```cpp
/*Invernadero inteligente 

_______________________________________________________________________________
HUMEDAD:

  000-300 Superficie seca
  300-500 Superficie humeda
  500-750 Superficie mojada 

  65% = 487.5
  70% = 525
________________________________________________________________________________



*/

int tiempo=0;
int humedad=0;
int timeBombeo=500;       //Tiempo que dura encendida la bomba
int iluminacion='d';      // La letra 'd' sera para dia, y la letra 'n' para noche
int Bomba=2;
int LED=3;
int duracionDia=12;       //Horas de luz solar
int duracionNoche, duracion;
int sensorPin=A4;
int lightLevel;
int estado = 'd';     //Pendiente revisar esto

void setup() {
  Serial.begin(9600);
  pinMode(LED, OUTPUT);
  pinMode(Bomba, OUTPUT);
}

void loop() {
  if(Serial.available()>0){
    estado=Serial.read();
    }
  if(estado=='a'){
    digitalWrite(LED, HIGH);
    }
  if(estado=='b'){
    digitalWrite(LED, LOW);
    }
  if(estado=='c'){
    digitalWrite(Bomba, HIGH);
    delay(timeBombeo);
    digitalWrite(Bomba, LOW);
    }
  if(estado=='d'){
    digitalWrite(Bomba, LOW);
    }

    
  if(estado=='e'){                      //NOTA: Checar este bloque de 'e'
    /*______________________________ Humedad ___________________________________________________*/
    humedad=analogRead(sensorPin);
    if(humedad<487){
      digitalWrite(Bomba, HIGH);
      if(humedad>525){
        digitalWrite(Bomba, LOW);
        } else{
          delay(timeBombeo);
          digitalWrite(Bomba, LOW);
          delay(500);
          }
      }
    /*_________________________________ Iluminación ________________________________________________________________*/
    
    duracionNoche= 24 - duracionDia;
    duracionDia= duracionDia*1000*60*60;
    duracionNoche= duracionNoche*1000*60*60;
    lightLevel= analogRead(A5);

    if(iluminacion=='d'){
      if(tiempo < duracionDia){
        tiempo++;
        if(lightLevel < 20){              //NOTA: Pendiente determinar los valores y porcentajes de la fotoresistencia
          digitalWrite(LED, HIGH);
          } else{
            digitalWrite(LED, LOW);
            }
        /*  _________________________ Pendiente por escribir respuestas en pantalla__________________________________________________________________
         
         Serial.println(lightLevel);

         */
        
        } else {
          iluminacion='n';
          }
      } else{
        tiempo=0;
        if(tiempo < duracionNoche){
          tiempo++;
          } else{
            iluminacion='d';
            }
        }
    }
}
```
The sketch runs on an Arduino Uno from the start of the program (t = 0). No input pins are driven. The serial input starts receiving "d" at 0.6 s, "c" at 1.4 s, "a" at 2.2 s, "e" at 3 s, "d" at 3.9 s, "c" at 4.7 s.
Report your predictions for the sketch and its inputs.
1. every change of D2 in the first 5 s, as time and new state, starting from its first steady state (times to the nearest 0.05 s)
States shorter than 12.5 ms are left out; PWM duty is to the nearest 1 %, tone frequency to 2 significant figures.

0 s low; 1.4 s high; 2.4 s low; 3 s high; 3.5 s low; 4.7 s high
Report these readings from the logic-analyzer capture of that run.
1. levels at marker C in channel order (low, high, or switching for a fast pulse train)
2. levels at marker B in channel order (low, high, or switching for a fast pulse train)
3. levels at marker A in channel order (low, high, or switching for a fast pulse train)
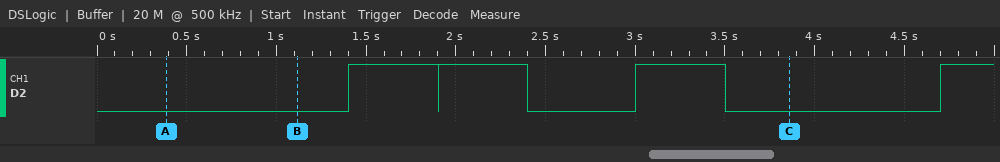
D2 low
D2 low
D2 low
